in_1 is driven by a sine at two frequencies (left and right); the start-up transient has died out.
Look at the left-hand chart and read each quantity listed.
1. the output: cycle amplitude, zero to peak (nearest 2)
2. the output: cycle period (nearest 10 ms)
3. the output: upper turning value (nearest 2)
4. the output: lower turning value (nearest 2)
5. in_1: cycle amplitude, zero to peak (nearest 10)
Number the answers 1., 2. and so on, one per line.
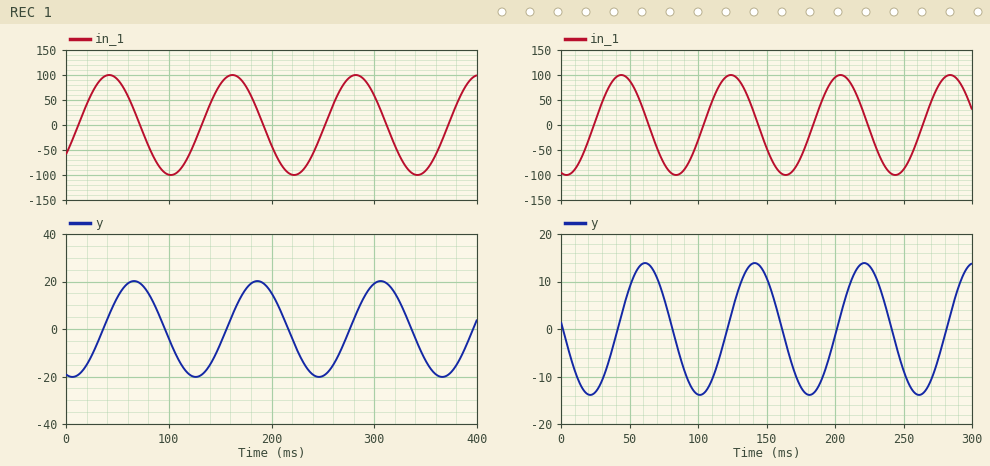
1. 20
2. 120 ms
3. 20
4. -20
5. 100
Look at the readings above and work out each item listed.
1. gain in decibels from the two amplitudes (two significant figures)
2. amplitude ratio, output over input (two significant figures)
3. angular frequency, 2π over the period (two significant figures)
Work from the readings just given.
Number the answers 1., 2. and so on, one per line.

1. -14 dB
2. 0.20
3. 0.052 rad/ms
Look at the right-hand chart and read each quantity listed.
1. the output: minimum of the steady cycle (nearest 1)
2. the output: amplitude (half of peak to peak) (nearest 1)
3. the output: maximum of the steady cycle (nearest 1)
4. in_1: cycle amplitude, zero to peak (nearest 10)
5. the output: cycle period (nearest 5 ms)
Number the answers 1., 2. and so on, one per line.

1. -14
2. 14
3. 14
4. 100
5. 80 ms
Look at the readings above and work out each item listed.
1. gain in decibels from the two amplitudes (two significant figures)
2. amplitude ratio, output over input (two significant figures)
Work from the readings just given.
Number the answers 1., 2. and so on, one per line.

1. -17 dB
2. 0.14
